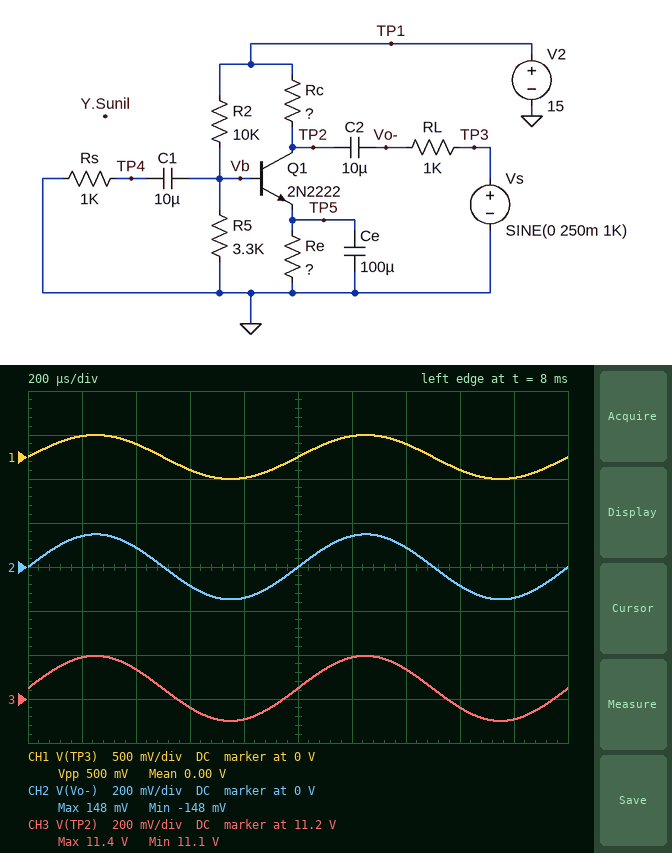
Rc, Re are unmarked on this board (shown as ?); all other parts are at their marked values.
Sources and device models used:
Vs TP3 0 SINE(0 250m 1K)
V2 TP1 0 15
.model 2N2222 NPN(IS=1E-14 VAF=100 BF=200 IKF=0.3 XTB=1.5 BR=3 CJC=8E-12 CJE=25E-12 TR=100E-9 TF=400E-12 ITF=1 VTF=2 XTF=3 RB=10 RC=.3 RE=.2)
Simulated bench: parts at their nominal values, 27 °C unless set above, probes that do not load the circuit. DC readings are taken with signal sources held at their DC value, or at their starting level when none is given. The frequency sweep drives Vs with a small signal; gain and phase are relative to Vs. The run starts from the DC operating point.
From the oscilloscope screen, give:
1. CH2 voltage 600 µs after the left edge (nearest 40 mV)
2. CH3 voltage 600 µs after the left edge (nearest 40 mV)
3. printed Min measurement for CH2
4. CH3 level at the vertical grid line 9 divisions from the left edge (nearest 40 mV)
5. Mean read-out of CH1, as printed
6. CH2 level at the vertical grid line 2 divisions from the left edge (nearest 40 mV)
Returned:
-80 mV
11.16 V
-148 mV
11.12 V
0.00 V
80 mV
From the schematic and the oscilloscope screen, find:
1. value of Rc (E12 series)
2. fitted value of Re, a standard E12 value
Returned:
1.5 kΩ
1.2 kΩ
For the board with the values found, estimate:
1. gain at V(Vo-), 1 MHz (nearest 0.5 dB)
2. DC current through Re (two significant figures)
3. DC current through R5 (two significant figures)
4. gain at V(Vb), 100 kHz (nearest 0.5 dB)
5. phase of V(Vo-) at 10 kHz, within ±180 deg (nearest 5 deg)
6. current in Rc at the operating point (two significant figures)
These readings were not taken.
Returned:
-7.0 dB
2.5 mA
1.1 mA
-63.0 dB
0 deg
2.5 mA
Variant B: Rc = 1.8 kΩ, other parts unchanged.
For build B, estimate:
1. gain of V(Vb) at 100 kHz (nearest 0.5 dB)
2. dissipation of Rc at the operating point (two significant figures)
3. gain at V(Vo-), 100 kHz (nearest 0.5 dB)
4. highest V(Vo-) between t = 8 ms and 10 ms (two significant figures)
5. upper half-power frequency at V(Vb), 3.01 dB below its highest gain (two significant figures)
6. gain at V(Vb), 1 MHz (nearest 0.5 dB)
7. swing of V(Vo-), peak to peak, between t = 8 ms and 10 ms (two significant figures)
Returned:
-62.0 dB
11 mW
-4.0 dB
160 mV
270 MHz
-45.0 dB
320 mV
